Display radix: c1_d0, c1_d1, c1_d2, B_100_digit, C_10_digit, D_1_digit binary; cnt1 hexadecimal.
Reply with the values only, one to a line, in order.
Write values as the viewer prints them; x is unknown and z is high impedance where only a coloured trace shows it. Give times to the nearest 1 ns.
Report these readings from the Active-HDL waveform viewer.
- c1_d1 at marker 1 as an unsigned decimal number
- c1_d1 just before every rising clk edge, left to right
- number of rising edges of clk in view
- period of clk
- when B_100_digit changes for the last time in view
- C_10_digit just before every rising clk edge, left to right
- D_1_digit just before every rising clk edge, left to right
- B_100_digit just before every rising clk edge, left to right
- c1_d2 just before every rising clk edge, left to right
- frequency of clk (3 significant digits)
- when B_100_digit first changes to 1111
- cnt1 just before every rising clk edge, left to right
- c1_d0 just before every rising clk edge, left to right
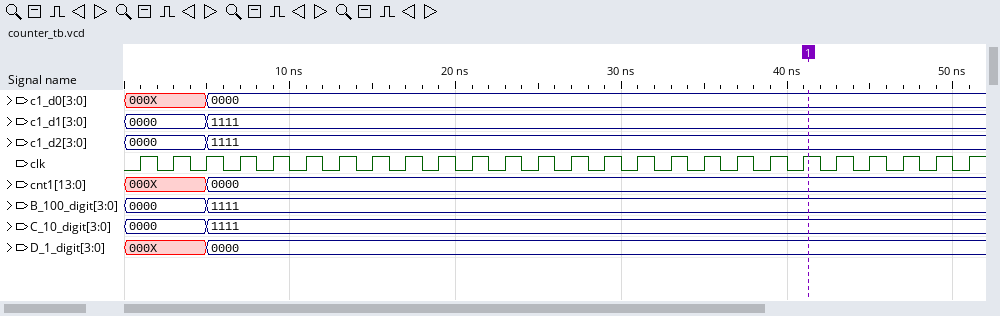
15
0000, 0000, 0000, 1111, 1111, 1111, 1111, 1111, 1111, 1111, 1111, 1111, 1111, 1111, 1111, 1111, 1111, 1111, 1111, 1111, 1111, 1111, 1111, 1111, 1111, 1111
26
2 ns
5 ns
0000, 0000, 0000, 1111, 1111, 1111, 1111, 1111, 1111, 1111, 1111, 1111, 1111, 1111, 1111, 1111, 1111, 1111, 1111, 1111, 1111, 1111, 1111, 1111, 1111, 1111
000X, 000X, 000X, 0000, 0000, 0000, 0000, 0000, 0000, 0000, 0000, 0000, 0000, 0000, 0000, 0000, 0000, 0000, 0000, 0000, 0000, 0000, 0000, 0000, 0000, 0000
0000, 0000, 0000, 1111, 1111, 1111, 1111, 1111, 1111, 1111, 1111, 1111, 1111, 1111, 1111, 1111, 1111, 1111, 1111, 1111, 1111, 1111, 1111, 1111, 1111, 1111
0000, 0000, 0000, 1111, 1111, 1111, 1111, 1111, 1111, 1111, 1111, 1111, 1111, 1111, 1111, 1111, 1111, 1111, 1111, 1111, 1111, 1111, 1111, 1111, 1111, 1111
500 MHz
5 ns
000X, 000X, 000X, 0000, 0000, 0000, 0000, 0000, 0000, 0000, 0000, 0000, 0000, 0000, 0000, 0000, 0000, 0000, 0000, 0000, 0000, 0000, 0000, 0000, 0000, 0000
000X, 000X, 000X, 0000, 0000, 0000, 0000, 0000, 0000, 0000, 0000, 0000, 0000, 0000, 0000, 0000, 0000, 0000, 0000, 0000, 0000, 0000, 0000, 0000, 0000, 0000
